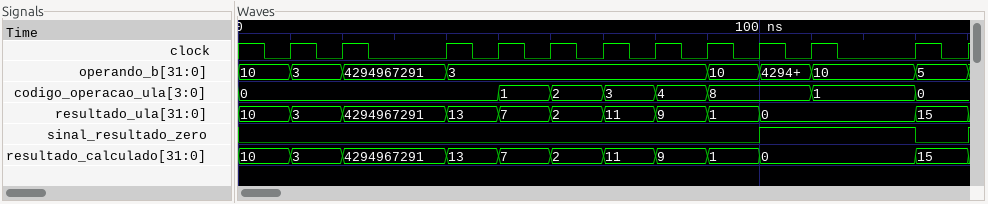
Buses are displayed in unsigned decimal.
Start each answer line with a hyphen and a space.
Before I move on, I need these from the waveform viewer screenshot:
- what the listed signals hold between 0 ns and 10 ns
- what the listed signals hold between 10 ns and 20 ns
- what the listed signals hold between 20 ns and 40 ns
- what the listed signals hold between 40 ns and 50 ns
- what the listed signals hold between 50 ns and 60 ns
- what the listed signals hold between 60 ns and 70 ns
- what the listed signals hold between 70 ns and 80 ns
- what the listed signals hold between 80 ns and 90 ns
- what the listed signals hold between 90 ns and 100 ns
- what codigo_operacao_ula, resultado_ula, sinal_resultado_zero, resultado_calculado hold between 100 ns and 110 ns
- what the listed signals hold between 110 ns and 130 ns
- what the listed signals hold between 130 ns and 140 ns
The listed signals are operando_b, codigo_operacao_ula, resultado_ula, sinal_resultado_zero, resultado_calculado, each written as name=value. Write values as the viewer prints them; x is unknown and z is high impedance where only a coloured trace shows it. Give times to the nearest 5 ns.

- operando_b=10, codigo_operacao_ula=0, resultado_ula=10, sinal_resultado_zero=0, resultado_calculado=10
- operando_b=3, codigo_operacao_ula=0, resultado_ula=3, sinal_resultado_zero=0, resultado_calculado=3
- operando_b=4294967291, codigo_operacao_ula=0, resultado_ula=4294967291, sinal_resultado_zero=0, resultado_calculado=4294967291
- operando_b=3, codigo_operacao_ula=0, resultado_ula=13, sinal_resultado_zero=0, resultado_calculado=13
- operando_b=3, codigo_operacao_ula=1, resultado_ula=7, sinal_resultado_zero=0, resultado_calculado=7
- operando_b=3, codigo_operacao_ula=2, resultado_ula=2, sinal_resultado_zero=0, resultado_calculado=2
- operando_b=3, codigo_operacao_ula=3, resultado_ula=11, sinal_resultado_zero=0, resultado_calculado=11
- operando_b=3, codigo_operacao_ula=4, resultado_ula=9, sinal_resultado_zero=0, resultado_calculado=9
- operando_b=10, codigo_operacao_ula=8, resultado_ula=1, sinal_resultado_zero=0, resultado_calculado=1
- codigo_operacao_ula=8, resultado_ula=0, sinal_resultado_zero=1, resultado_calculado=0
- operando_b=10, codigo_operacao_ula=1, resultado_ula=0, sinal_resultado_zero=1, resultado_calculado=0
- operando_b=5, codigo_operacao_ula=0, resultado_ula=15, sinal_resultado_zero=0, resultado_calculado=15
